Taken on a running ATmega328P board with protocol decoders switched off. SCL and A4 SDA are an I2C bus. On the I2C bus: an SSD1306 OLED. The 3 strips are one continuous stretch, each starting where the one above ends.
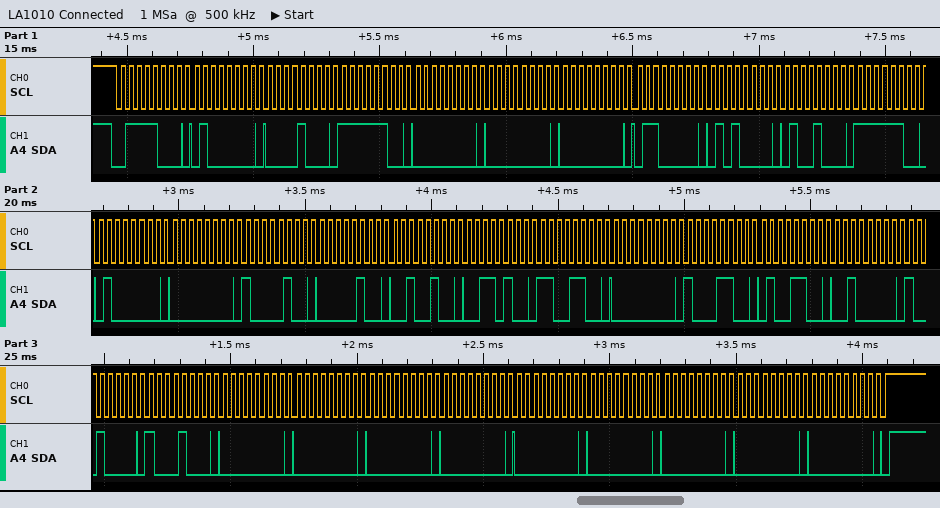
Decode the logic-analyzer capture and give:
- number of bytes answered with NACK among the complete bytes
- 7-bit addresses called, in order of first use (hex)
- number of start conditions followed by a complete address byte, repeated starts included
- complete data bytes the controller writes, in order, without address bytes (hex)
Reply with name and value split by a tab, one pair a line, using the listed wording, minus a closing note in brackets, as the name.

number of bytes answered with NACK among the complete bytes	0
7-bit addresses called, in order of first use	0x3C
number of start conditions followed by a complete address byte, repeated starts included	1
complete data bytes the controller writes, in order, without address bytes	40 08 FC 00 00 00 60 50 48 FC 40 00 84 04 24 34 CC 00 8C 4C 20 90 88 00 00 00 00 00 00 00 00 00
